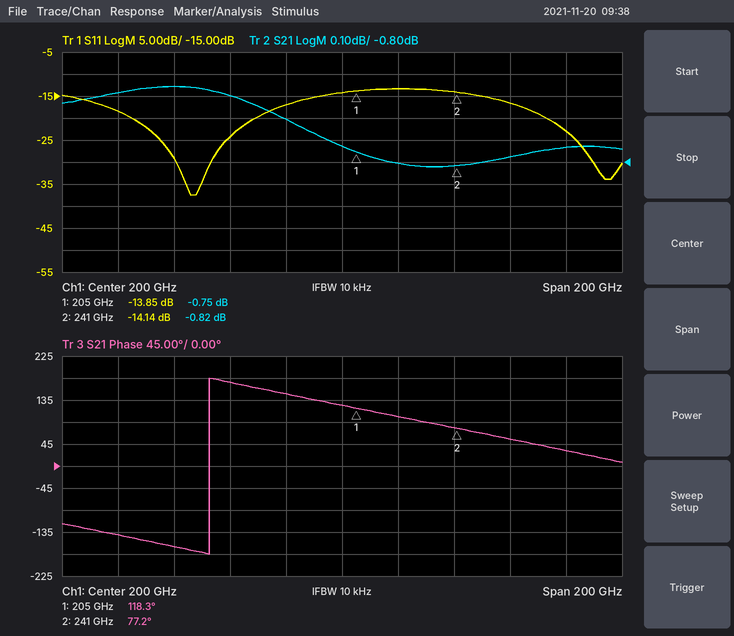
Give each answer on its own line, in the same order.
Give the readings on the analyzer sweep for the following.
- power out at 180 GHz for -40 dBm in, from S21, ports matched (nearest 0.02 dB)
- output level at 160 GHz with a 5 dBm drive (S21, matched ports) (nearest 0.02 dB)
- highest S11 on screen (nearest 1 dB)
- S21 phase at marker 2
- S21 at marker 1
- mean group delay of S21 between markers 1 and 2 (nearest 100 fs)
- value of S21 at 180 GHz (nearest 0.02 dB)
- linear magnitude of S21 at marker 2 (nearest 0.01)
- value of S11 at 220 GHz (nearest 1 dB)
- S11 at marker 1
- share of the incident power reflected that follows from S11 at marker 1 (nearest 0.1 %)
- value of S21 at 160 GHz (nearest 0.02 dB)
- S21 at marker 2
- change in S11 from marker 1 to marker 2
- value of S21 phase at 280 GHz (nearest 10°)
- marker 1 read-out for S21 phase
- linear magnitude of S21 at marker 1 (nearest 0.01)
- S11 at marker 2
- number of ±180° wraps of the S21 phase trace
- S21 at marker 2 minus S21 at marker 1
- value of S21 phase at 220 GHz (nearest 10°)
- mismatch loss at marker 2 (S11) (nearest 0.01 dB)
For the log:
-40.60 dBm
4.50 dBm
-13 dB
77.2°
-0.75 dB
3.2 ps
-0.60 dB
0.91
-13 dB
-13.85 dB
4.1 %
-0.50 dB
-0.82 dB
-0.29 dB
30°
118.3°
0.92
-14.14 dB
1
-0.07 dB
100°
0.17 dB
